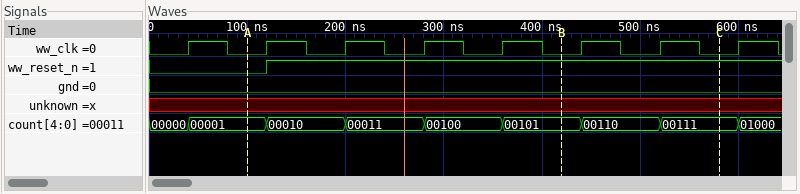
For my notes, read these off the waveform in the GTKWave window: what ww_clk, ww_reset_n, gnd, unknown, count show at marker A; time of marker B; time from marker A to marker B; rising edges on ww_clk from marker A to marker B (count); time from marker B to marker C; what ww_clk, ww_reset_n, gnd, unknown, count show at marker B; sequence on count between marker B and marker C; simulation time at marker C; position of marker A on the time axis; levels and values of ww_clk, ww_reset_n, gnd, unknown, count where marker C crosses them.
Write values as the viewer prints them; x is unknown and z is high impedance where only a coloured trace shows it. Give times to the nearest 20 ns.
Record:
ww_clk=0, ww_reset_n=0, gnd=0, unknown=x, count=00001
420 ns
320 ns
4
160 ns
ww_clk=0, ww_reset_n=1, gnd=0, unknown=x, count=00101
00101, 00110, 00111
580 ns
100 ns
ww_clk=0, ww_reset_n=1, gnd=0, unknown=x, count=00111
